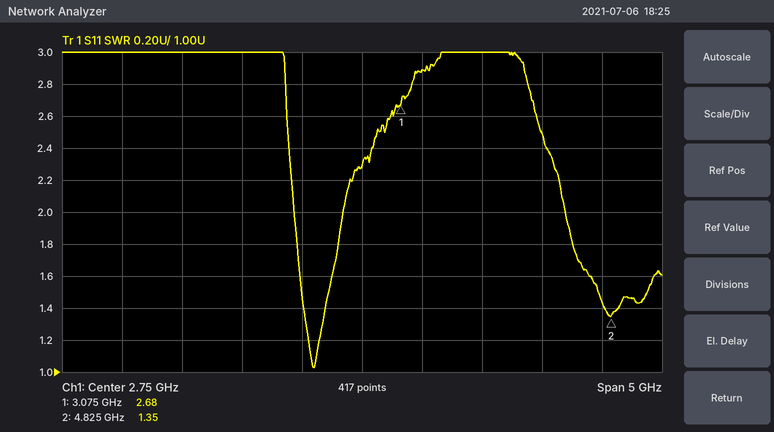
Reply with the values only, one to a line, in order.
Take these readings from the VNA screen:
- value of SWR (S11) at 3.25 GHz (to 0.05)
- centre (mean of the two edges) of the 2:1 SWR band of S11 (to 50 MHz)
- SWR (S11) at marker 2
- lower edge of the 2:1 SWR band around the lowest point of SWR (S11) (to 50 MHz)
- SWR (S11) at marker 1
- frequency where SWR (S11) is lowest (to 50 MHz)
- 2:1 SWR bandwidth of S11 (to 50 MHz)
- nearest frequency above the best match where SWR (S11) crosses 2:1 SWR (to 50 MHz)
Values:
2.90
2.40 GHz
1.35
2.20 GHz
2.68
2.35 GHz
400 MHz
2.60 GHz
